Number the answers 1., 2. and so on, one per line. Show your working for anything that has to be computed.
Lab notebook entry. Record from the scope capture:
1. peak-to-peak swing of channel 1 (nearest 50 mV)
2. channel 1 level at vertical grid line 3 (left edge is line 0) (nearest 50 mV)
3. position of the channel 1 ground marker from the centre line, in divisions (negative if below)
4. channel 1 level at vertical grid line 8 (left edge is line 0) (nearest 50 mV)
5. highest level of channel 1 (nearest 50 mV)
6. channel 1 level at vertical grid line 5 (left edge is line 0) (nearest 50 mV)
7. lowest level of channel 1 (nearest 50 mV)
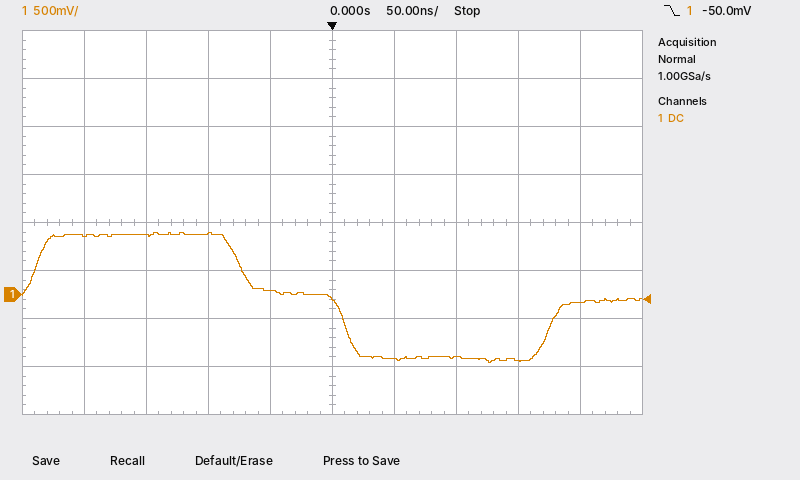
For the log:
1. 650 mV − (-700 mV) = 1.35 V
2. 650 mV
3. -1.5 div
4. -700 mV
5. 650 mV
6. -50 mV
7. -700 mV
